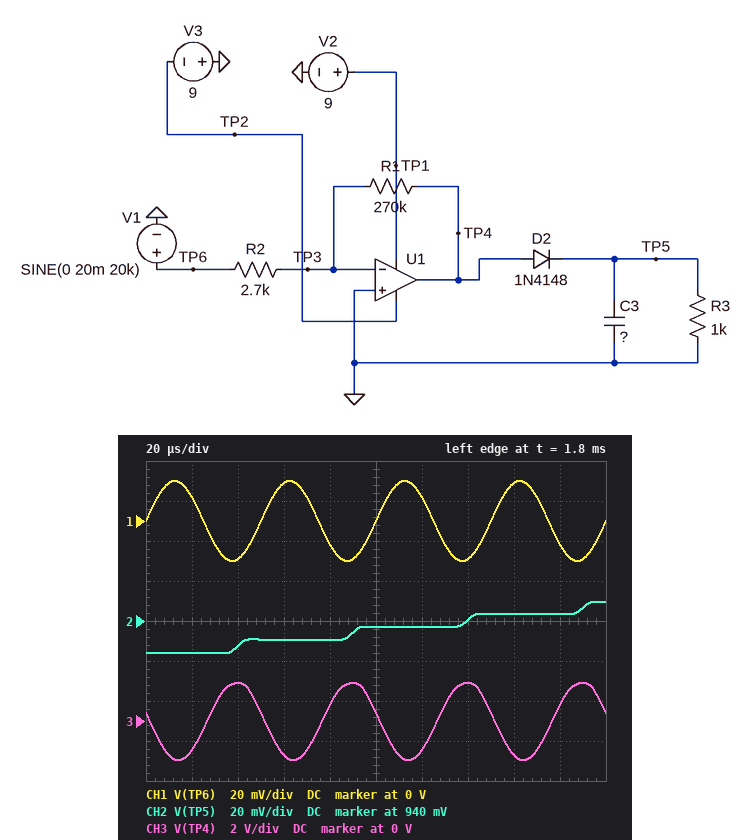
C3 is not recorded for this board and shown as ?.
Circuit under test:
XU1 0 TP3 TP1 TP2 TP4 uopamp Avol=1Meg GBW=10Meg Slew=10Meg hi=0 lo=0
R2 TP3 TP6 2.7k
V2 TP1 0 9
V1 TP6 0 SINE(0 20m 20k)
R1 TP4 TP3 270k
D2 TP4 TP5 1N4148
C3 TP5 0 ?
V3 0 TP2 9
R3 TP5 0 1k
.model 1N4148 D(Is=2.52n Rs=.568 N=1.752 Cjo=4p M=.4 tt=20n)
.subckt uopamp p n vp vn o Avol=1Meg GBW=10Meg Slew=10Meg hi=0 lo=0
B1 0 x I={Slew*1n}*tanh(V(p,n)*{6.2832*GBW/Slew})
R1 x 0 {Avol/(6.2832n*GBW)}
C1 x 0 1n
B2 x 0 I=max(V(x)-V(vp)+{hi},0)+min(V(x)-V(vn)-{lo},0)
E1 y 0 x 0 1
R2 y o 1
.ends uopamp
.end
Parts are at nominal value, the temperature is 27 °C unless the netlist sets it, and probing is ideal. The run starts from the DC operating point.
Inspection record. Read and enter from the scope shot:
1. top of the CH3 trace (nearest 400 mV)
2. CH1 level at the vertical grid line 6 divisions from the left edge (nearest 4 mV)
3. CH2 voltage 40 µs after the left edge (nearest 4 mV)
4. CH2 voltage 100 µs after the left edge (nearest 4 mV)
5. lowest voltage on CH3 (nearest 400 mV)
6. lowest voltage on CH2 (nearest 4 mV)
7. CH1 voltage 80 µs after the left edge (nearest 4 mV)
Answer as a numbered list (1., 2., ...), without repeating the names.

1. 2.0 V
2. 12 mV
3. 928 mV
4. 936 mV
5. -2.0 V
6. 924 mV
7. -12 mV
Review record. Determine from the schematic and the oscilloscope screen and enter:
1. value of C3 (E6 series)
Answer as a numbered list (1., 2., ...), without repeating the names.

1. 220 µF
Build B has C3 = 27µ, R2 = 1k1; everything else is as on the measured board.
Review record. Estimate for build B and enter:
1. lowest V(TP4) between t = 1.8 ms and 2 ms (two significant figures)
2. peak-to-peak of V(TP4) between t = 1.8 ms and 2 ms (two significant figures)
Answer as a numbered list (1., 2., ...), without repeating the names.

1. -4.4 V
2. 8.8 V
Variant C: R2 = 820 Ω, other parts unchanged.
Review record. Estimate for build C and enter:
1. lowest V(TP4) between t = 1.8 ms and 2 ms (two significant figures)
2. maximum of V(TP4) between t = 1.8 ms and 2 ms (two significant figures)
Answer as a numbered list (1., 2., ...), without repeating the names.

1. -5.5 V
2. 5.1 V
